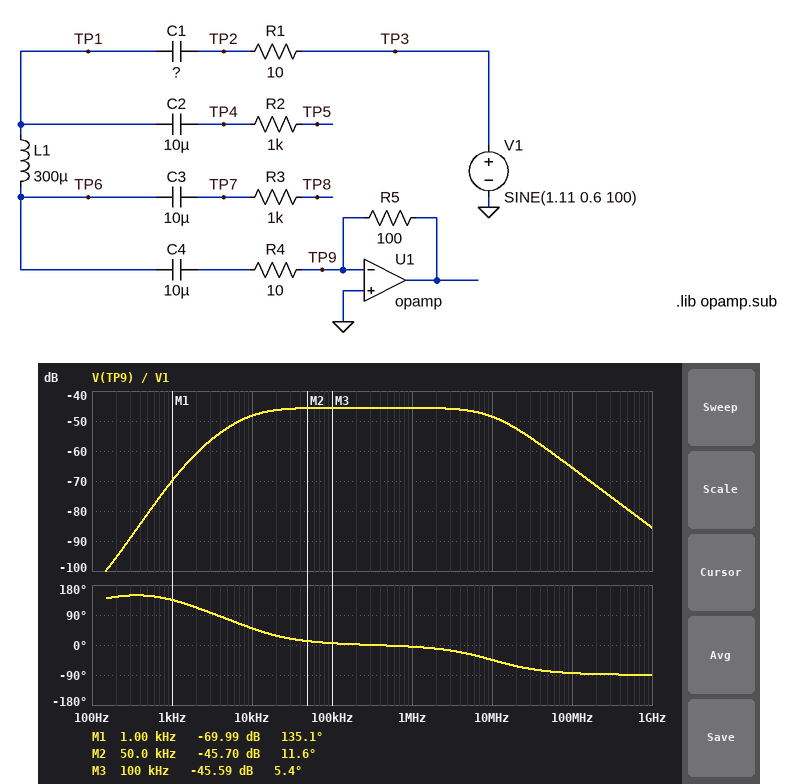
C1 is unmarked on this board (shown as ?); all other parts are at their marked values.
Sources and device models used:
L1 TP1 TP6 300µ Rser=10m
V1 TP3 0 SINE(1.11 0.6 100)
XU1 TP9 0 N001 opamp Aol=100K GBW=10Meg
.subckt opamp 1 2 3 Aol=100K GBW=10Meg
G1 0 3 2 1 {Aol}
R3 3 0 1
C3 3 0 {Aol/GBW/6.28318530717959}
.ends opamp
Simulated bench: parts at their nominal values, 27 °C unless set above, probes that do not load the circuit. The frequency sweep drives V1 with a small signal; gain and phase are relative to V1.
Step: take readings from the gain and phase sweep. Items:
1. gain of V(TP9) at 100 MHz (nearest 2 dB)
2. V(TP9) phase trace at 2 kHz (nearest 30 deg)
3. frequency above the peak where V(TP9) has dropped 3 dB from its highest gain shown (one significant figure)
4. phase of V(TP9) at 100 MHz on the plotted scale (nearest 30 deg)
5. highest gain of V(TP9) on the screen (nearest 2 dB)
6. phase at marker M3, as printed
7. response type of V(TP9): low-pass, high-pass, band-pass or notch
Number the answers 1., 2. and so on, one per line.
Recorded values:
1. -66 dB
2. 120 deg
3. 10 MHz
4. -90 deg
5. -46 dB
6. 5.4 deg
7. band-pass
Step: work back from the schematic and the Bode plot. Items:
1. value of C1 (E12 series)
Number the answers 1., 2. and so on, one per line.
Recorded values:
1. 15 µF
